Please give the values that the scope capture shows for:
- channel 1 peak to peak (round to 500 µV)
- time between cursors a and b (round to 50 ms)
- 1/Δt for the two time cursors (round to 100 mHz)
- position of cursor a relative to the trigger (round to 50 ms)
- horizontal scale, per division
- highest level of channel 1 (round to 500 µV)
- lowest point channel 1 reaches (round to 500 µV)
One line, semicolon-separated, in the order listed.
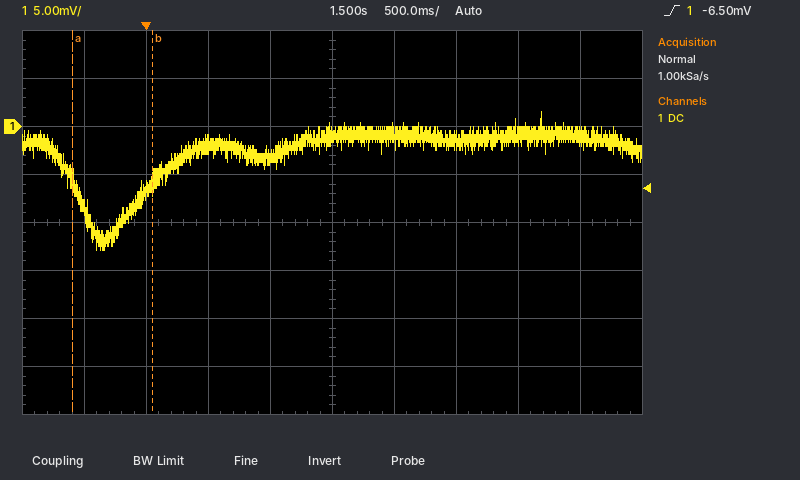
14.5 mV; 650 ms; 1.5 Hz; -600 ms; 500 ms; 1.5 mV; -13.0 mV
